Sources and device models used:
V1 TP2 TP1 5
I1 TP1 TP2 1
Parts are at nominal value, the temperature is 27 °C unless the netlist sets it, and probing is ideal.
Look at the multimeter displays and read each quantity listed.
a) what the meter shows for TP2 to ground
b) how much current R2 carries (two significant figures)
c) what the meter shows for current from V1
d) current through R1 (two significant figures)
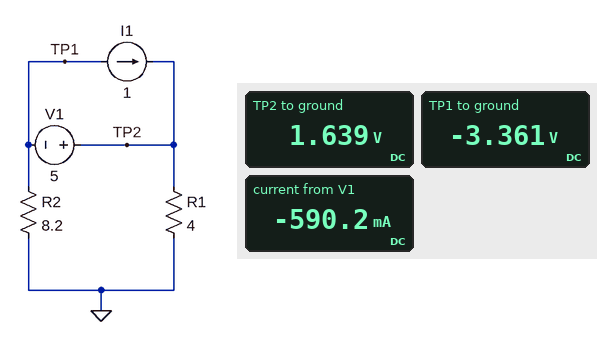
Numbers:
1.639 V
410 mA
-590.2 mA
410 mA
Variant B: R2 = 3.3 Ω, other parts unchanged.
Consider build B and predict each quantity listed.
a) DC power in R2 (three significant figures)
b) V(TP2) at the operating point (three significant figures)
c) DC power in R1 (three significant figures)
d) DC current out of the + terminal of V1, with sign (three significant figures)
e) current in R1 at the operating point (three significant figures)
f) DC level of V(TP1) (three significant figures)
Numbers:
1.55 W
2.74 V
1.88 W
-315 mA
685 mA
-2.26 V
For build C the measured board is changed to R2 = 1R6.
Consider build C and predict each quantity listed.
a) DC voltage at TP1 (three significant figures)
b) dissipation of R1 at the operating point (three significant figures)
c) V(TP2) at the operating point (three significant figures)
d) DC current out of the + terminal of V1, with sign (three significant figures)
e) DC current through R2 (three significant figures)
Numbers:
-1.43 V
3.19 W
3.57 V
-107 mA
893 mA
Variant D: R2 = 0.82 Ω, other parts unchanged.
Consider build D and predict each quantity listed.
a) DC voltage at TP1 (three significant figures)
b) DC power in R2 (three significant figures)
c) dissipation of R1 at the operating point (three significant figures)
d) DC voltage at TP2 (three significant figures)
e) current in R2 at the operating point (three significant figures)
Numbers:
-851 mV
882 mW
4.30 W
4.15 V
1.04 A
